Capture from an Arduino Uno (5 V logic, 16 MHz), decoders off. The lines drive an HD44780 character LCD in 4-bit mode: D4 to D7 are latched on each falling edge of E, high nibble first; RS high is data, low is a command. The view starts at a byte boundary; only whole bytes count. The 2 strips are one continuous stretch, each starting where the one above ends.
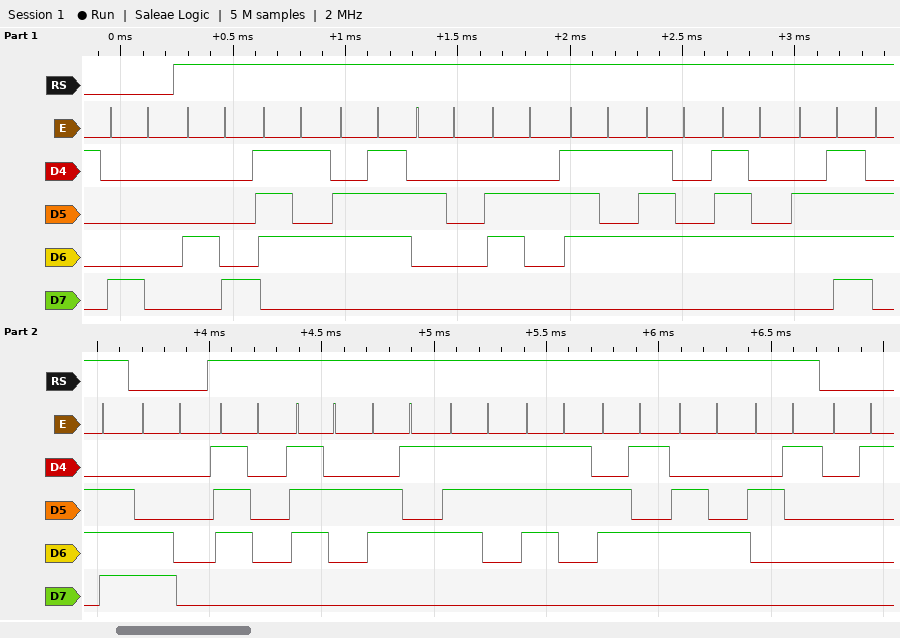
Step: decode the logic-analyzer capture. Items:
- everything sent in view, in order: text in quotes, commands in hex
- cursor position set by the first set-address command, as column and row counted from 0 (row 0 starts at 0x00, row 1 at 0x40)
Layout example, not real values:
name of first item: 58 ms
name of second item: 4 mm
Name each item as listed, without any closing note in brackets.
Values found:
everything sent in view, in order: text in quotes, commands in hex: 0x80 "Hug button" 0xC0 "pressed!" 0x01
cursor position set by the first set-address command, as column and row counted from 0: column 0, row 0
